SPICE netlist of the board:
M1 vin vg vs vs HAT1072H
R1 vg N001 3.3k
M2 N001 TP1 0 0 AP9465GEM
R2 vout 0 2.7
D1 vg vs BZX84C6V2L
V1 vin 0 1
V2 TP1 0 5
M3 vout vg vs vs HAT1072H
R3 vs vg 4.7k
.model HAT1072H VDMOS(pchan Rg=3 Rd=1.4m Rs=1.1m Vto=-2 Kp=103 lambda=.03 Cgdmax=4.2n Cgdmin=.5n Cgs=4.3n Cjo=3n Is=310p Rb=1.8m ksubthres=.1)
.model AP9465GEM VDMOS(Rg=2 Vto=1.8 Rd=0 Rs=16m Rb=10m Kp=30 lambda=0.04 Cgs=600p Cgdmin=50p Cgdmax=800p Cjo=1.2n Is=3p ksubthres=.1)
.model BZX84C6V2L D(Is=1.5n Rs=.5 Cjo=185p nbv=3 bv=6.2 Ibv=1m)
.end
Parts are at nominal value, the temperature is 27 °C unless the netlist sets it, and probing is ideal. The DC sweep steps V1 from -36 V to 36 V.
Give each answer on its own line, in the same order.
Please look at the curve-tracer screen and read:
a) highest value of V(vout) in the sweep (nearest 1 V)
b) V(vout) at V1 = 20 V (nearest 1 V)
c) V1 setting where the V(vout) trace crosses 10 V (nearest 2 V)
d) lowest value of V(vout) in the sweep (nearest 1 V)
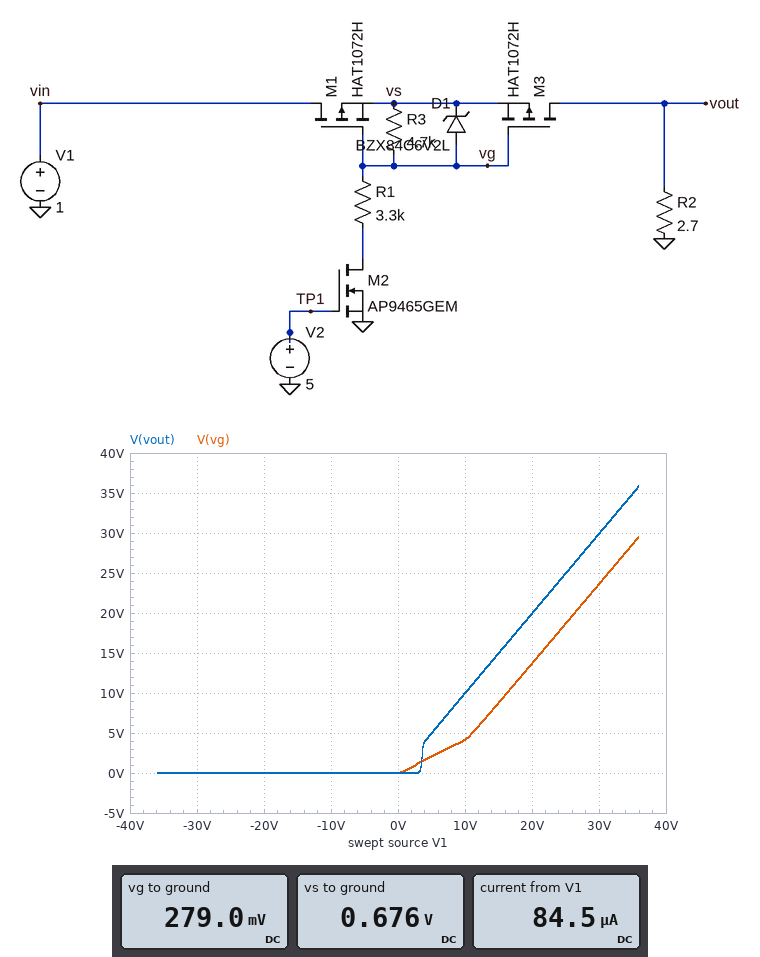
36 V
20 V
10 V
0 V
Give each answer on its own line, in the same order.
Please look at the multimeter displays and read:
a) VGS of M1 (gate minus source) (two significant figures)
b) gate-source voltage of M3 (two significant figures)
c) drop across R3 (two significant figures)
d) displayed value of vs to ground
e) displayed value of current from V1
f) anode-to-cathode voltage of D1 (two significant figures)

-400 mV
-400 mV
400 mV
0.676 V
84.5 µA
-400 mV
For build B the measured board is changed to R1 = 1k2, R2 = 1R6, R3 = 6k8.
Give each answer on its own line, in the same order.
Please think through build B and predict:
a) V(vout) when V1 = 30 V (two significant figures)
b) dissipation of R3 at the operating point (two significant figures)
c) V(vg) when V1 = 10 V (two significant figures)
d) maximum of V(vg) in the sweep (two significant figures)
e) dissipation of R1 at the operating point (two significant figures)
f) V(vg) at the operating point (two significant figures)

30 V
49 µW
3.7 V
29 V
8.6 µW
100 mV
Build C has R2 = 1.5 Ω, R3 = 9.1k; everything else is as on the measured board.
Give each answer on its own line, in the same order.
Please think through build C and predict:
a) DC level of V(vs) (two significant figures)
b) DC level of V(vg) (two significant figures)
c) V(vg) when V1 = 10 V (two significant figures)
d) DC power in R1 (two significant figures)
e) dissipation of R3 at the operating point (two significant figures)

690 mV
180 mV
3.8 V
10 µW
28 µW
